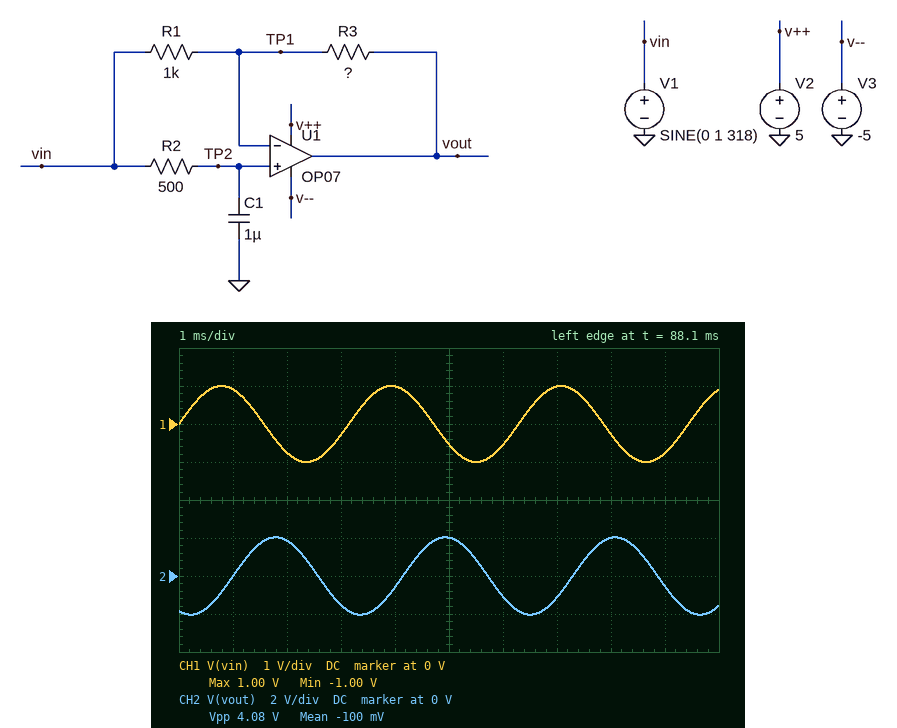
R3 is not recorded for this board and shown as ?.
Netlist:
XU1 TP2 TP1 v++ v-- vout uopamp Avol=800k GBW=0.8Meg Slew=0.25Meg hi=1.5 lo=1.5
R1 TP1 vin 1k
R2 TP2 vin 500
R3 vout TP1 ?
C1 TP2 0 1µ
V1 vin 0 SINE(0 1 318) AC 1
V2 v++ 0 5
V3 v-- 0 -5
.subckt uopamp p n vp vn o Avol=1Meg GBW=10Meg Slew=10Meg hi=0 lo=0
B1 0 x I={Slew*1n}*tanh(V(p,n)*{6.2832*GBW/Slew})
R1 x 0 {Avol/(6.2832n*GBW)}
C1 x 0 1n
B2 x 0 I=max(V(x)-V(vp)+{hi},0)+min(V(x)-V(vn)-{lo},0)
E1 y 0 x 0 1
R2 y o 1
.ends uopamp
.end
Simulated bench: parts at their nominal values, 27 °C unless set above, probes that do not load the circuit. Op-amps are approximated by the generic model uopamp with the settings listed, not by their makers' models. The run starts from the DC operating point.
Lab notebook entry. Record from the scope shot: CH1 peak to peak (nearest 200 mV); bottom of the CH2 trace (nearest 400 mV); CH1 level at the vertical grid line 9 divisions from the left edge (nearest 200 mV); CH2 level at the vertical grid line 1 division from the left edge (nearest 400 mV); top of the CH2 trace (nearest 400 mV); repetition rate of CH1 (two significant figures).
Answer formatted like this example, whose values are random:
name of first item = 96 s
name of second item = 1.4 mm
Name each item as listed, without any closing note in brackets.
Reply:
CH1 peak to peak = 2.0 V
bottom of the CH2 trace = -2.0 V
CH1 level at the vertical grid line 9 divisions from the left edge = -800 mV
CH2 level at the vertical grid line 1 division from the left edge = 0 V
top of the CH2 trace = 2.0 V
repetition rate of CH1 = 320 Hz
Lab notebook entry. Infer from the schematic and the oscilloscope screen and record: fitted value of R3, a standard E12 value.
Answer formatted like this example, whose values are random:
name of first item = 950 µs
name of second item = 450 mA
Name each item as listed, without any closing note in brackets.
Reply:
fitted value of R3, a standard E12 value = 2.7 kΩ
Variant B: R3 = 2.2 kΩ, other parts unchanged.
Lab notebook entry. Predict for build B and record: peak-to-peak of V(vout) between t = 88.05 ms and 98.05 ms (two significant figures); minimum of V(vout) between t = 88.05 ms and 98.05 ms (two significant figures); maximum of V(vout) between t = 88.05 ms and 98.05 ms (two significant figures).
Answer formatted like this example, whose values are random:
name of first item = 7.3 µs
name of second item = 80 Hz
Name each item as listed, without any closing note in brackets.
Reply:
peak-to-peak of V(vout) between t = 88.05 ms and 98.05 ms = 3.4 V
minimum of V(vout) between t = 88.05 ms and 98.05 ms = -1.7 V
maximum of V(vout) between t = 88.05 ms and 98.05 ms = 1.7 V
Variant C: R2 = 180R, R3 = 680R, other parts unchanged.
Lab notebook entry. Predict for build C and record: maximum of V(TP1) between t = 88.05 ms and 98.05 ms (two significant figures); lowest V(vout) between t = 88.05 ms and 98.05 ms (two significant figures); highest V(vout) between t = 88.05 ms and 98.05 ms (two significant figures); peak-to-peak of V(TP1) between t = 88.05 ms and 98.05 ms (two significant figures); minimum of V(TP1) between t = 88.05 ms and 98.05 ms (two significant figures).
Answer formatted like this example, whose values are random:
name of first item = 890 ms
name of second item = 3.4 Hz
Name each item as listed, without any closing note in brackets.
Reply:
maximum of V(TP1) between t = 88.05 ms and 98.05 ms = 940 mV
lowest V(vout) between t = 88.05 ms and 98.05 ms = -970 mV
highest V(vout) between t = 88.05 ms and 98.05 ms = 970 mV
peak-to-peak of V(TP1) between t = 88.05 ms and 98.05 ms = 1.9 V
minimum of V(TP1) between t = 88.05 ms and 98.05 ms = -940 mV
